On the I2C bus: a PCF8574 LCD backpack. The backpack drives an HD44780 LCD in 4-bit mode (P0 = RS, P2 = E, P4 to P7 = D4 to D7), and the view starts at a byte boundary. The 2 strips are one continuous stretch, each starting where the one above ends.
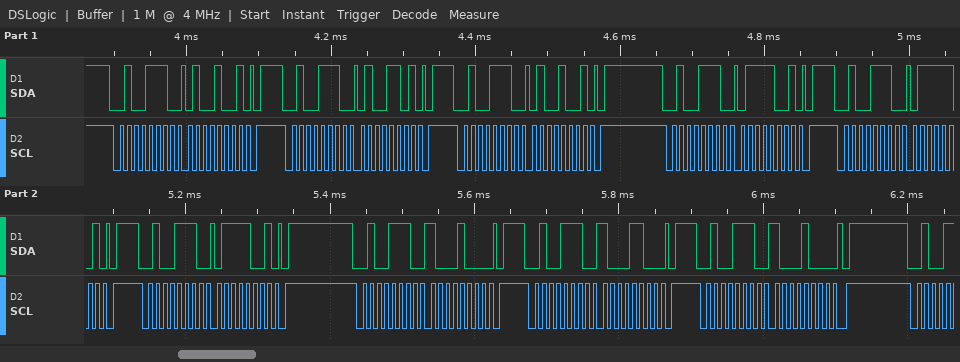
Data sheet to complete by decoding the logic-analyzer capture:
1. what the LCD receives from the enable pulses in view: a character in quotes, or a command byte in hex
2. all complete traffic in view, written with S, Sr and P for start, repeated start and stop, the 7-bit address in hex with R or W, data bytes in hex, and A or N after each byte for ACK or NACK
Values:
'G'
S 27W A 49 A P S 27W A 4D A P S 27W A 49 A P S 27W A 79 A P S 27W A 7D A P S 27W A 79 A P S 27W A 88 A P S 27W A 8C A P S 27W A 88 A P
